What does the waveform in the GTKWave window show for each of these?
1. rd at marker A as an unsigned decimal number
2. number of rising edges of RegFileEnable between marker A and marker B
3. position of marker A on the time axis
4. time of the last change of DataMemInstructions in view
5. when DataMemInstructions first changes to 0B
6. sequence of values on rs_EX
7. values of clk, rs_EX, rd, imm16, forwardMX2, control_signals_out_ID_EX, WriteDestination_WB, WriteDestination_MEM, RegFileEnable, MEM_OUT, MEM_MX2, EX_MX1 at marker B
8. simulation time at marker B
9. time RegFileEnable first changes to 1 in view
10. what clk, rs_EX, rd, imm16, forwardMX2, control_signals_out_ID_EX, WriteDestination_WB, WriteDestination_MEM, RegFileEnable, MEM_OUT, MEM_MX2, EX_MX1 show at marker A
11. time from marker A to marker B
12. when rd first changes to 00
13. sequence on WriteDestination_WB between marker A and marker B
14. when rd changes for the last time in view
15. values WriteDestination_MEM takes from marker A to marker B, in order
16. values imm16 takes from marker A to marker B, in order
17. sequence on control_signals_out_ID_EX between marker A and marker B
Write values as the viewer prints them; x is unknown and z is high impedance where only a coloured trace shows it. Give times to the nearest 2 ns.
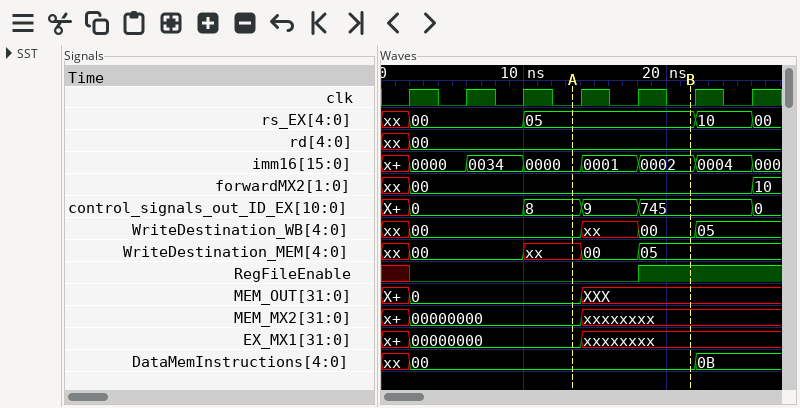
0
1
14 ns
22 ns
22 ns
xx, 00, 05, 10, 00
clk=0, rs_EX=05, rd=00, imm16=0002, forwardMX2=00, control_signals_out_ID_EX=745, WriteDestination_WB=00, WriteDestination_MEM=05, RegFileEnable=1, MEM_OUT=XXX, MEM_MX2=xxxxxxxx, EX_MX1=xxxxxxxx
22 ns
18 ns
clk=0, rs_EX=05, rd=00, imm16=0000, forwardMX2=00, control_signals_out_ID_EX=8, WriteDestination_WB=00, WriteDestination_MEM=xx, RegFileEnable=0, MEM_OUT=0, MEM_MX2=00000000, EX_MX1=00000000
8 ns
2 ns
00, xx, 00
2 ns
xx, 00, 05
0000, 0001, 0002
8, 9, 745
